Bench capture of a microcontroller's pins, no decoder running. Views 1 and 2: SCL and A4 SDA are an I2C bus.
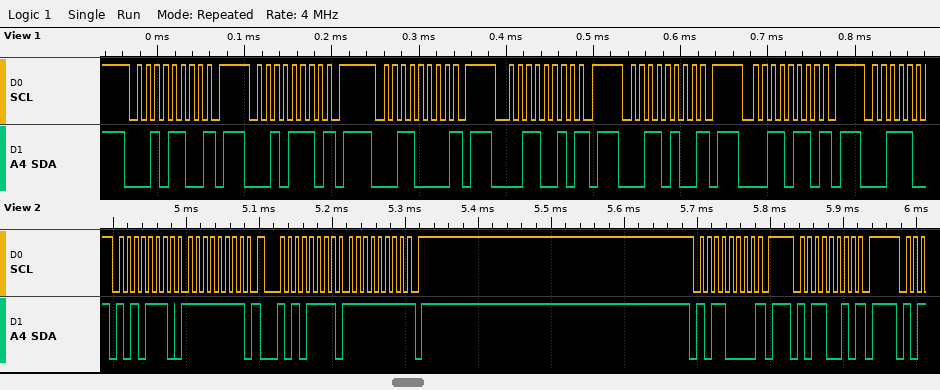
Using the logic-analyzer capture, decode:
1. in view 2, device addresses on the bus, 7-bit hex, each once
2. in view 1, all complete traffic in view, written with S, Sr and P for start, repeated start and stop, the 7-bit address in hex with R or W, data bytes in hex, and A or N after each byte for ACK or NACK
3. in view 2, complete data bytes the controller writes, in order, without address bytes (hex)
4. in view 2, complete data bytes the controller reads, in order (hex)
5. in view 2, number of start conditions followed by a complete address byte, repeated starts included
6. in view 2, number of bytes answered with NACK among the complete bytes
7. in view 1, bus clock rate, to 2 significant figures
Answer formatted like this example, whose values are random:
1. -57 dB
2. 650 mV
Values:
1. 0x57 0x58 0x59
2. S 16W N P S 17W N P S 18W N P S 19W N P S 1AW N P S 1BW N P
3. FF
4. FF
5. 4
6. 3
7. 100 kHz
